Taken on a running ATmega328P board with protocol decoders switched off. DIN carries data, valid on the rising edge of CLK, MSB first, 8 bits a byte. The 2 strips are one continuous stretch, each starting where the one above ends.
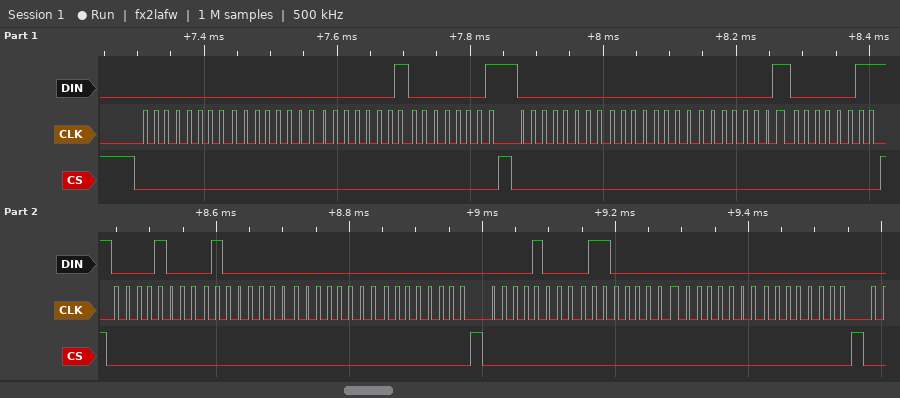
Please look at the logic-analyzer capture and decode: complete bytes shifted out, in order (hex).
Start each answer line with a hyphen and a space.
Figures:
- 00 00 01 01 00 00 01 03 08 40 00 00 08 60 00 00
